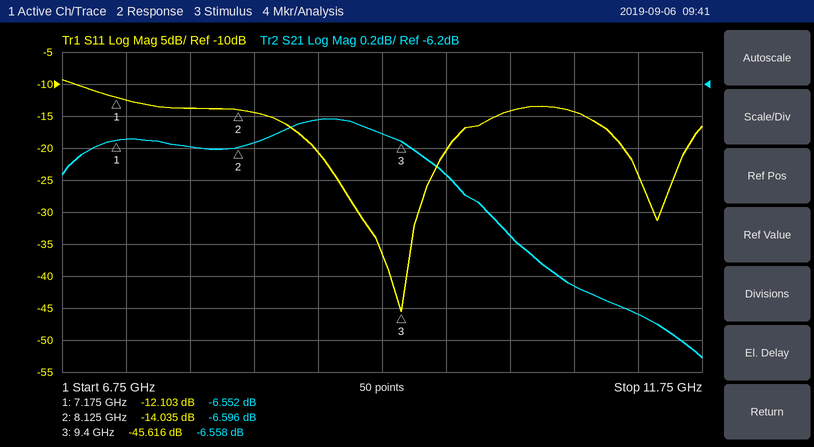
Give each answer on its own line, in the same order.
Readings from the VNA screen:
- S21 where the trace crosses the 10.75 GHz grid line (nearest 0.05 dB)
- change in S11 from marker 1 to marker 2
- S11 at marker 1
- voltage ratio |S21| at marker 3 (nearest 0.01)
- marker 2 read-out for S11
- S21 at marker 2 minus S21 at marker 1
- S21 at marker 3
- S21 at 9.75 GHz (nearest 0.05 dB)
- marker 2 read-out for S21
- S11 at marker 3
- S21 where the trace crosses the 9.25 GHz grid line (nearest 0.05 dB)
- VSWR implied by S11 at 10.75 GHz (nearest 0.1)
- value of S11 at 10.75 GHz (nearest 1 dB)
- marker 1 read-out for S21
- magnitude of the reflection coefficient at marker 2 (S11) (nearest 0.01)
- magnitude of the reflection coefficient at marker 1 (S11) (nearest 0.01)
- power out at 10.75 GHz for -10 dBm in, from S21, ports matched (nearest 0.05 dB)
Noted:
-7.45 dB
-1.932 dB
-12.103 dB
0.47
-14.035 dB
-0.044 dB
-6.558 dB
-6.75 dB
-6.596 dB
-45.616 dB
-6.50 dB
1.5
-14 dB
-6.552 dB
0.20
0.25
-17.45 dBm
